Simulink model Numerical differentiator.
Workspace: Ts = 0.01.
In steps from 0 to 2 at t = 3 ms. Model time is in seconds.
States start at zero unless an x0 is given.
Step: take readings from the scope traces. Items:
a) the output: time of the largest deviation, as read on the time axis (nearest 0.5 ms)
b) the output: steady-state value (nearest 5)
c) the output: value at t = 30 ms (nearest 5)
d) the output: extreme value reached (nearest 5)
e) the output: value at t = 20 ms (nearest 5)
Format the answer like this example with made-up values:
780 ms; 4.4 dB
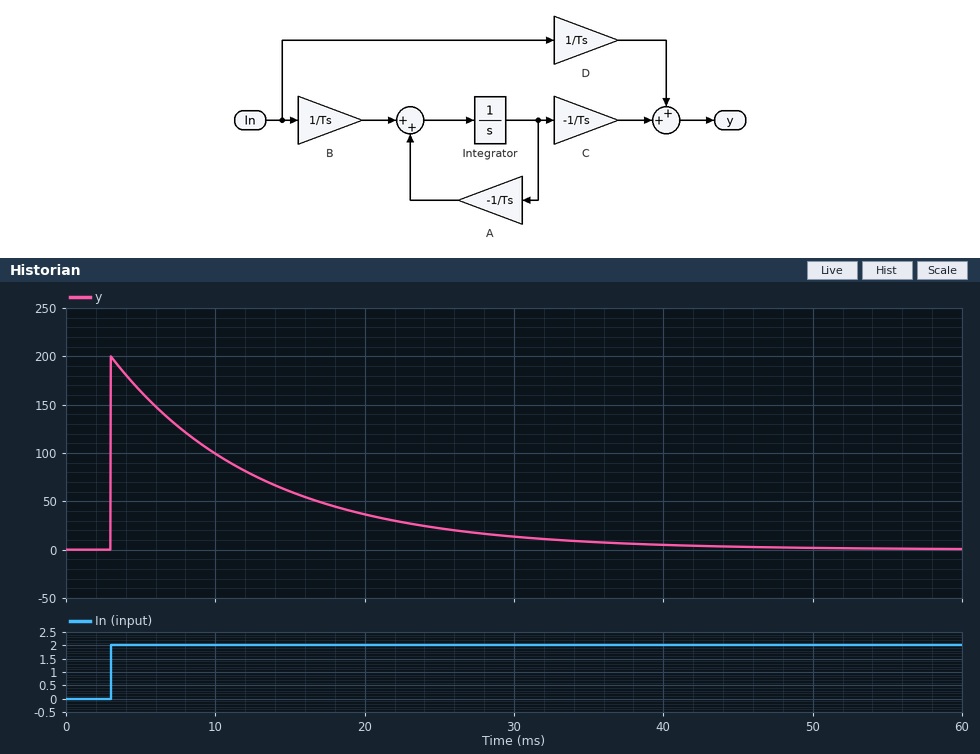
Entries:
3.0 ms; 0; 15; 200; 35
